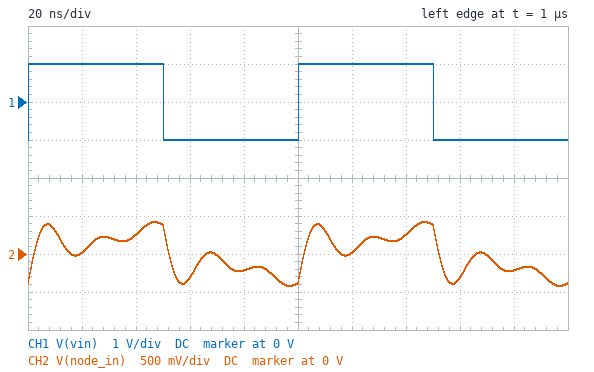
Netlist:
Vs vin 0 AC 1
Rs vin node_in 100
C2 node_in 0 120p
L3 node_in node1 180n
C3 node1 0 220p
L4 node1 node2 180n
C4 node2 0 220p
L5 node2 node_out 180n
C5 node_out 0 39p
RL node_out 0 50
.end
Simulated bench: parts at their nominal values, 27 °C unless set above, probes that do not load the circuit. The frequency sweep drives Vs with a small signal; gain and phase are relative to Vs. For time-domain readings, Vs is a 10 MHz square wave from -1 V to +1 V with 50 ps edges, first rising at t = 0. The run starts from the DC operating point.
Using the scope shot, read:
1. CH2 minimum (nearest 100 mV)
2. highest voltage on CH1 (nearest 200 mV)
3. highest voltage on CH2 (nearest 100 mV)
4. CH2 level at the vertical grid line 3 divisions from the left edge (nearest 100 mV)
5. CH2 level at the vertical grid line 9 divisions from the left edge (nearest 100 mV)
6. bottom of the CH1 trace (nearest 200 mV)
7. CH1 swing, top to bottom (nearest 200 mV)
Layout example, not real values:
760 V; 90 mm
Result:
-400 mV; 1.0 V; 400 mV; -300 mV; -200 mV; -1.0 V; 2.0 V
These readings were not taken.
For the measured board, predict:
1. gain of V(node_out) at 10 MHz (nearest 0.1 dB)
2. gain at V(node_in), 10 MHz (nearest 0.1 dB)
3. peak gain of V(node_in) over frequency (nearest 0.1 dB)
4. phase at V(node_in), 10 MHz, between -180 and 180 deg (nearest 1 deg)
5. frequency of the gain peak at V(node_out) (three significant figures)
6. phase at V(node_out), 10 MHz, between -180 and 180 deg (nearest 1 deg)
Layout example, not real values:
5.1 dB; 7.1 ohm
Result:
-11.6 dB; -14.3 dB; -2.1 dB; -24 deg; 29.4 MHz; -72 deg
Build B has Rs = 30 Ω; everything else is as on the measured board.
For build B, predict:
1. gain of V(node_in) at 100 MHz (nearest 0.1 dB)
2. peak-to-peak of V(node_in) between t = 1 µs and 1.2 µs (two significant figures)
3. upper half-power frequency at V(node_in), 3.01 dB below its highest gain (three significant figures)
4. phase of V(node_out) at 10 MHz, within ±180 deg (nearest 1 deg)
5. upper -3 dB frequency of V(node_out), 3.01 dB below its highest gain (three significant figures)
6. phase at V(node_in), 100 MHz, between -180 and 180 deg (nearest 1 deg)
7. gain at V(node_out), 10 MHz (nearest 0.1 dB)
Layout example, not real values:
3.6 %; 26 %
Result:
-6.9 dB; 1.4 V; 69.7 MHz; -64 deg; 46.3 MHz; -63 deg; -4.2 dB
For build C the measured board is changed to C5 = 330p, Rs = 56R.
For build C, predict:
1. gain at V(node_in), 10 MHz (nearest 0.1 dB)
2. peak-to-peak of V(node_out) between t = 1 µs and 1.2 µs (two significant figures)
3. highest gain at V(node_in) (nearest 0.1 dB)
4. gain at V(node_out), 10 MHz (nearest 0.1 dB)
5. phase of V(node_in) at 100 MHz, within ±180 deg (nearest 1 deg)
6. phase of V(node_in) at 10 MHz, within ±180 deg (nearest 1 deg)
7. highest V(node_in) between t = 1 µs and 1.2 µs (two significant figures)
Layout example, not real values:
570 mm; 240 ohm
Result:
-13.7 dB; 950 mV; -0.2 dB; -8.4 dB; -75 deg; 9 deg; 530 mV
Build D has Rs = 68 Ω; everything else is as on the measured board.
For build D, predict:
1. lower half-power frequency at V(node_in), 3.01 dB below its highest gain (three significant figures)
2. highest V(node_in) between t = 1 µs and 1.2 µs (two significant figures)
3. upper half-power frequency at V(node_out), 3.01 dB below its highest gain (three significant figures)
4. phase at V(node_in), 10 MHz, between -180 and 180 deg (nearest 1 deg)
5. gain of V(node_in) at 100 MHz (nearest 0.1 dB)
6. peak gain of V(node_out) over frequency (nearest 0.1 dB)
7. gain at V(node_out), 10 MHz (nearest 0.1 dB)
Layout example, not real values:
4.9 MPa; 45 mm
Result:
45.5 MHz; 520 mV; 48.0 MHz; -22 deg; -13.2 dB; -7.4 dB; -8.9 dB
